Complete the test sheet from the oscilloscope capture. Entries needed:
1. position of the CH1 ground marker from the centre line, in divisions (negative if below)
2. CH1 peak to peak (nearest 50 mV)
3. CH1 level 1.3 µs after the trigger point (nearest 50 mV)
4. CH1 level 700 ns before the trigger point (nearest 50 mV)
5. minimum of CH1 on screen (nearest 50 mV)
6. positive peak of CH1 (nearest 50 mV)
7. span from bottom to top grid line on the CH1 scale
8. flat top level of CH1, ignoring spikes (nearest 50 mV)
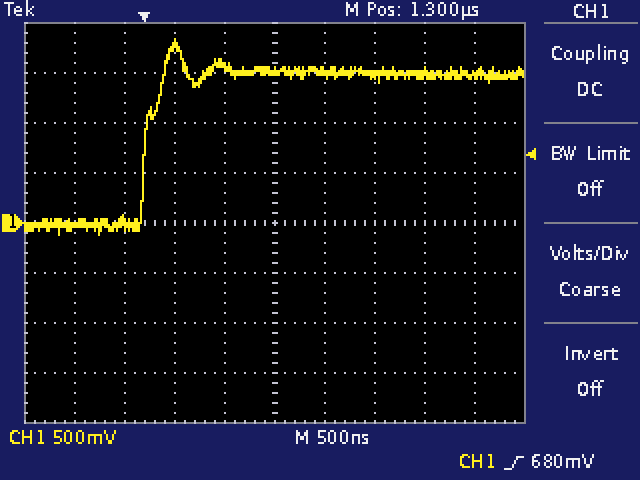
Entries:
0.0 div
1.95 V
1.50 V
-50 mV
-100 mV
1.85 V
4 V
1.50 V
